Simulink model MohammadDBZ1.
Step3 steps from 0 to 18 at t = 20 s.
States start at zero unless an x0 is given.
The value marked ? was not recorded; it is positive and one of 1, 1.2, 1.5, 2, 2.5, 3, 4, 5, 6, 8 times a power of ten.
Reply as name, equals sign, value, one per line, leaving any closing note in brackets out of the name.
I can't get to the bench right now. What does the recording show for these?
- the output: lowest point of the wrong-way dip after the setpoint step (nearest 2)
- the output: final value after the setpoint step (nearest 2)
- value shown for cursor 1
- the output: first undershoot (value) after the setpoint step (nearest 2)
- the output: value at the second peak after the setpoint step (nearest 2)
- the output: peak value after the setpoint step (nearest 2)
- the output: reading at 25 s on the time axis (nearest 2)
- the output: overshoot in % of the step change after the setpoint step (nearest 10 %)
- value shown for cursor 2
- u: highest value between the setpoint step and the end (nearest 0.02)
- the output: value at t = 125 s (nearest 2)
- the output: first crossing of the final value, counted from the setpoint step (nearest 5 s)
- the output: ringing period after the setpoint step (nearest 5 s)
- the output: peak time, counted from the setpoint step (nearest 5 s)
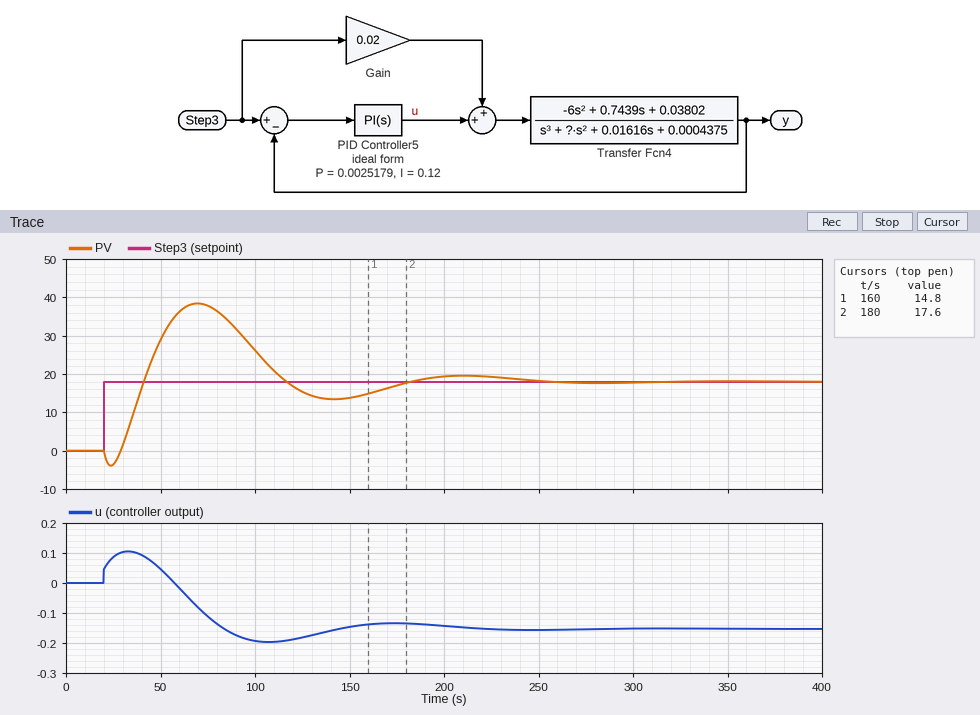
the output: lowest point of the wrong-way dip after the setpoint step = -4
the output: final value after the setpoint step = 18
value shown for cursor 1 = 14.8
the output: first undershoot (value) after the setpoint step = 14
the output: value at the second peak after the setpoint step = 20
the output: peak value after the setpoint step = 38
the output: reading at 25 s on the time axis = -4
the output: overshoot in % of the step change after the setpoint step = 110 %
value shown for cursor 2 = 17.6
u: highest value between the setpoint step and the end = 0.10
the output: value at t = 125 s = 16
the output: first crossing of the final value, counted from the setpoint step = 20 s
the output: ringing period after the setpoint step = 140 s
the output: peak time, counted from the setpoint step = 50 s
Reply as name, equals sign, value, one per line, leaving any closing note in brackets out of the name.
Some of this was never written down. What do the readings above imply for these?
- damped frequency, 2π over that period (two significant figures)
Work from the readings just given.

damped frequency, 2π over that period = 0.045 rad/s
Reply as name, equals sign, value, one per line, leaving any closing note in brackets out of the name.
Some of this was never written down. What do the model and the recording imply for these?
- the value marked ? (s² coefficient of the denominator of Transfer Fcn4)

the value marked ? = 0.3
